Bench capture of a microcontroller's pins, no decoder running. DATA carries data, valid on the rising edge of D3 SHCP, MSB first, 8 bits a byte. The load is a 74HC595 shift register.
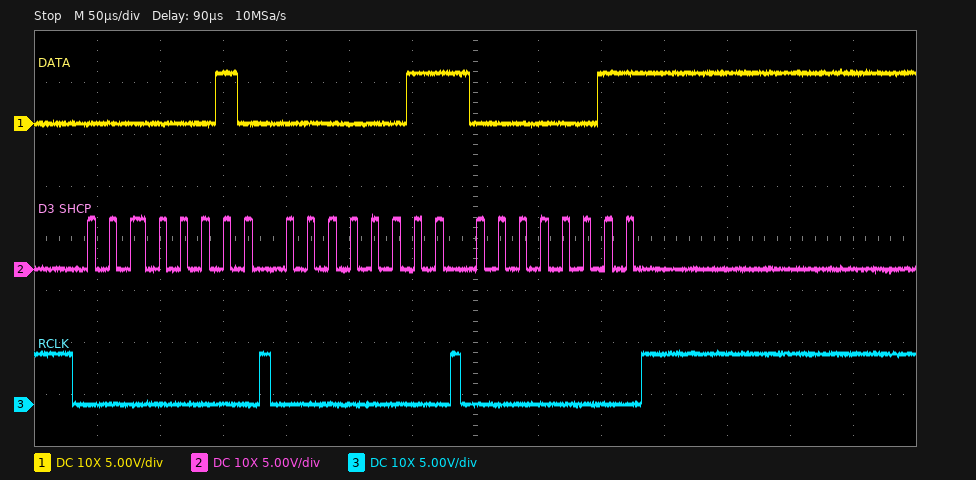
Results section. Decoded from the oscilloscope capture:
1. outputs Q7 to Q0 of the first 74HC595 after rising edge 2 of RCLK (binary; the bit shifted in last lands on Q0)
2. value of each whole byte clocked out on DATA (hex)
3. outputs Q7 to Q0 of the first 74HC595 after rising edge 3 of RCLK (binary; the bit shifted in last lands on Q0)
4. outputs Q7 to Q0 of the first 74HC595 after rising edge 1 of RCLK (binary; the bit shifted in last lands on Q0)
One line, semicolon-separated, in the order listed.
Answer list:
00000011; 02 03 03; 00000011; 00000010
